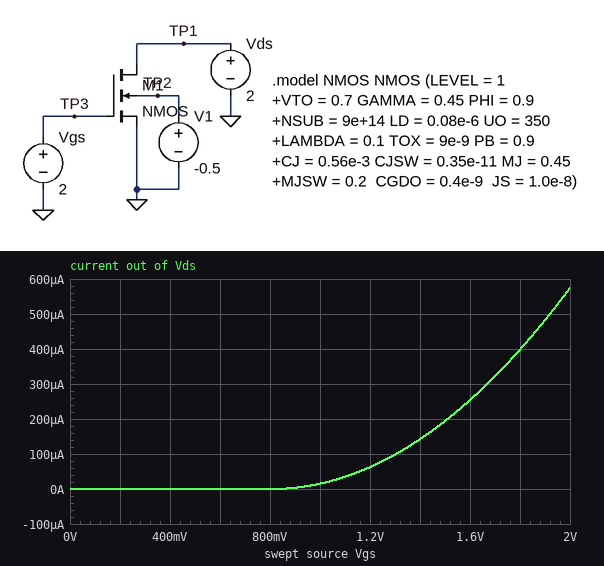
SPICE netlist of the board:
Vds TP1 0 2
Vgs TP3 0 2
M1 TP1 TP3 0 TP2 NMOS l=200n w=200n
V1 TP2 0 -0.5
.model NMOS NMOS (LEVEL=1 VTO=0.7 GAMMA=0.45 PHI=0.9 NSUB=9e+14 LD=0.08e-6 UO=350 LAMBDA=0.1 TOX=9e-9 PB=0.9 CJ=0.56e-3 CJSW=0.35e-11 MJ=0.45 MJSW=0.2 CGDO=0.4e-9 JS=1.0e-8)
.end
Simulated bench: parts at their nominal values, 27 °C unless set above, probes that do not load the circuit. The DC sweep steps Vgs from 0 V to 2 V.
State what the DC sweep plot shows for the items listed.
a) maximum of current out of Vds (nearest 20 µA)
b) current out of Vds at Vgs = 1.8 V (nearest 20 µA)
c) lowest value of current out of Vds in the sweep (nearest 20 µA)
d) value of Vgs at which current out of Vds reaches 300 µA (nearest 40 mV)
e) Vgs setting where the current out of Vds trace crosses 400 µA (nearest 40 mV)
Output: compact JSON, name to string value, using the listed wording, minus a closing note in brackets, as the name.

{"maximum of current out of Vds": "580 µA", "current out of Vds at Vgs = 1.8 V": "400 µA", "lowest value of current out of Vds in the sweep": "0 A", "value of Vgs at which current out of Vds reaches 300 µA": "1.68 V", "Vgs setting where the current out of Vds trace crosses 400 µA": "1.80 V"}
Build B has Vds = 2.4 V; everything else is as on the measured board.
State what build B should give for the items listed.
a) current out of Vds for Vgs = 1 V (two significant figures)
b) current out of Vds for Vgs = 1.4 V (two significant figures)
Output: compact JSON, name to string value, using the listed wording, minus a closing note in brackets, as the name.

{"current out of Vds for Vgs = 1 V": "16 µA", "current out of Vds for Vgs = 1.4 V": "150 µA"}
